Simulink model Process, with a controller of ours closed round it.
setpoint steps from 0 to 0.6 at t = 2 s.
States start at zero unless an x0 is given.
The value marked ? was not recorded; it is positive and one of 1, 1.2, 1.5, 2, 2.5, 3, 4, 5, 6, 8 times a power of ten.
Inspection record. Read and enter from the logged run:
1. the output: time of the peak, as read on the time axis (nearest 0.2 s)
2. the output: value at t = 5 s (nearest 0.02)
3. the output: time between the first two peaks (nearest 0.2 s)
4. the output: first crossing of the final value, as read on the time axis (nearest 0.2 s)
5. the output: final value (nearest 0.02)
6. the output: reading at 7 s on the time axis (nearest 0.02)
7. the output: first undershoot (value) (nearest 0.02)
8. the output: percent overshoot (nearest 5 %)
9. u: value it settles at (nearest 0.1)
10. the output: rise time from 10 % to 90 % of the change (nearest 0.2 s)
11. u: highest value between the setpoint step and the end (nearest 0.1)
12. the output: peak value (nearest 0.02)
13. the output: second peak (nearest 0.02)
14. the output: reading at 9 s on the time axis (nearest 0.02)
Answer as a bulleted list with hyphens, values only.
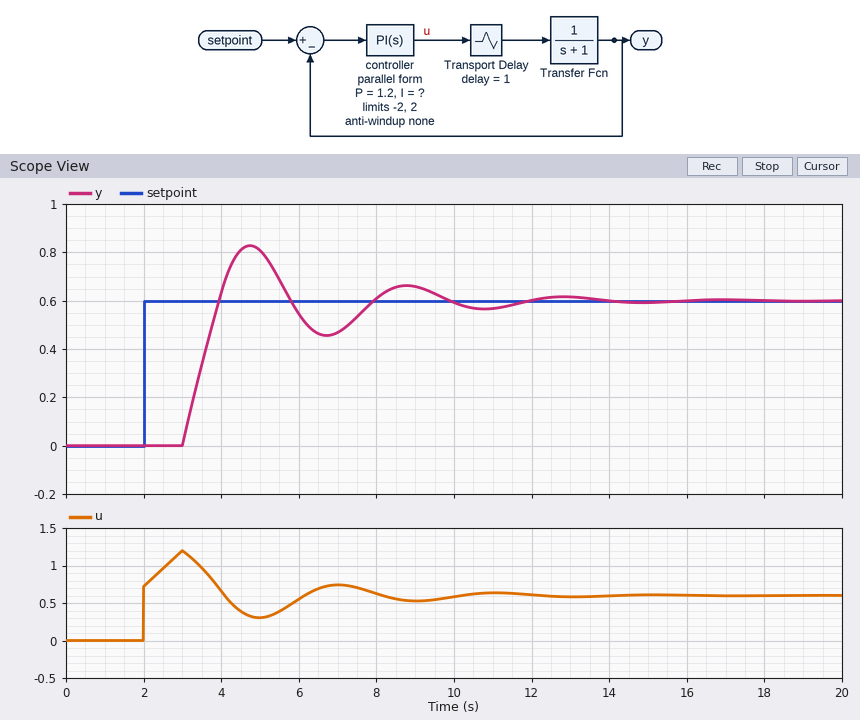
- 4.8 s
- 0.80
- 4.0 s
- 4.0 s
- 0.60
- 0.46
- 0.46
- 40 %
- 0.6
- 0.8 s
- 1.2
- 0.82
- 0.66
- 0.66
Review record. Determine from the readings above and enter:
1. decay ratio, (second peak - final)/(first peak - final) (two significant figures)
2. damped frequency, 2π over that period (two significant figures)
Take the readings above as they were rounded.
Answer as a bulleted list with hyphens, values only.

- 0.27
- 1.6 rad/s
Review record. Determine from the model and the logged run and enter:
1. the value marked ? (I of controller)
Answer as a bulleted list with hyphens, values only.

- 0.8
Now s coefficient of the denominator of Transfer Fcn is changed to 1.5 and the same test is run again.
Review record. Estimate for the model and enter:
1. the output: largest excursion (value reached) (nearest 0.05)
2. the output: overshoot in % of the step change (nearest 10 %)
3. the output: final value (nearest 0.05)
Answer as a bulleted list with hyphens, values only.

- 0.80
- 30 %
- 0.60
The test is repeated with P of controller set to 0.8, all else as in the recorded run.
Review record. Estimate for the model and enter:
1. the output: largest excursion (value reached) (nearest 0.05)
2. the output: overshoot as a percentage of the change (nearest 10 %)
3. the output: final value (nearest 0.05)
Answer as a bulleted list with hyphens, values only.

- 0.80
- 30 %
- 0.60
